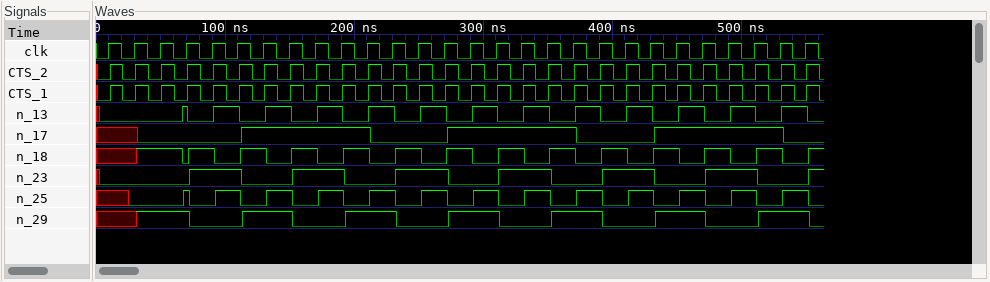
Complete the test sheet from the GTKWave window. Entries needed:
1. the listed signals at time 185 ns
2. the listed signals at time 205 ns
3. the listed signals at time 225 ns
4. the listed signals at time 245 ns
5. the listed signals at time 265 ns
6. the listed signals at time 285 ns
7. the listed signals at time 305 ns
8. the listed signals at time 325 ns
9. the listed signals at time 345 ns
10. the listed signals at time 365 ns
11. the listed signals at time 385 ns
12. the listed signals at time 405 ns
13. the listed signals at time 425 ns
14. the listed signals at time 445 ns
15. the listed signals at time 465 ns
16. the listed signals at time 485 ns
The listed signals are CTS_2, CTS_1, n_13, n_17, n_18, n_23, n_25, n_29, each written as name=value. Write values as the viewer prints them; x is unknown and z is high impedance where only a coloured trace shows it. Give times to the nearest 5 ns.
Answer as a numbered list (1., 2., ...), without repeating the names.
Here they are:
1. CTS_2=0, CTS_1=0, n_13=1, n_17=1, n_18=0, n_23=1, n_25=1, n_29=0
2. CTS_2=0, CTS_1=0, n_13=0, n_17=1, n_18=1, n_23=0, n_25=0, n_29=1
3. CTS_2=0, CTS_1=0, n_13=1, n_17=0, n_18=0, n_23=0, n_25=1, n_29=1
4. CTS_2=0, CTS_1=0, n_13=0, n_17=0, n_18=1, n_23=1, n_25=0, n_29=0
5. CTS_2=0, CTS_1=0, n_13=1, n_17=0, n_18=0, n_23=1, n_25=1, n_29=0
6. CTS_2=0, CTS_1=0, n_13=0, n_17=1, n_18=1, n_23=0, n_25=0, n_29=1
7. CTS_2=0, CTS_1=0, n_13=1, n_17=1, n_18=0, n_23=0, n_25=1, n_29=1
8. CTS_2=0, CTS_1=0, n_13=0, n_17=1, n_18=1, n_23=1, n_25=0, n_29=0
9. CTS_2=0, CTS_1=0, n_13=1, n_17=1, n_18=0, n_23=1, n_25=1, n_29=0
10. CTS_2=0, CTS_1=0, n_13=0, n_17=1, n_18=1, n_23=0, n_25=0, n_29=1
11. CTS_2=0, CTS_1=0, n_13=1, n_17=0, n_18=0, n_23=0, n_25=1, n_29=1
12. CTS_2=0, CTS_1=0, n_13=0, n_17=0, n_18=1, n_23=1, n_25=0, n_29=0
13. CTS_2=0, CTS_1=0, n_13=1, n_17=0, n_18=0, n_23=1, n_25=1, n_29=0
14. CTS_2=0, CTS_1=0, n_13=0, n_17=1, n_18=1, n_23=0, n_25=0, n_29=1
15. CTS_2=0, CTS_1=0, n_13=1, n_17=1, n_18=0, n_23=0, n_25=1, n_29=1
16. CTS_2=0, CTS_1=0, n_13=0, n_17=1, n_18=1, n_23=1, n_25=0, n_29=0
